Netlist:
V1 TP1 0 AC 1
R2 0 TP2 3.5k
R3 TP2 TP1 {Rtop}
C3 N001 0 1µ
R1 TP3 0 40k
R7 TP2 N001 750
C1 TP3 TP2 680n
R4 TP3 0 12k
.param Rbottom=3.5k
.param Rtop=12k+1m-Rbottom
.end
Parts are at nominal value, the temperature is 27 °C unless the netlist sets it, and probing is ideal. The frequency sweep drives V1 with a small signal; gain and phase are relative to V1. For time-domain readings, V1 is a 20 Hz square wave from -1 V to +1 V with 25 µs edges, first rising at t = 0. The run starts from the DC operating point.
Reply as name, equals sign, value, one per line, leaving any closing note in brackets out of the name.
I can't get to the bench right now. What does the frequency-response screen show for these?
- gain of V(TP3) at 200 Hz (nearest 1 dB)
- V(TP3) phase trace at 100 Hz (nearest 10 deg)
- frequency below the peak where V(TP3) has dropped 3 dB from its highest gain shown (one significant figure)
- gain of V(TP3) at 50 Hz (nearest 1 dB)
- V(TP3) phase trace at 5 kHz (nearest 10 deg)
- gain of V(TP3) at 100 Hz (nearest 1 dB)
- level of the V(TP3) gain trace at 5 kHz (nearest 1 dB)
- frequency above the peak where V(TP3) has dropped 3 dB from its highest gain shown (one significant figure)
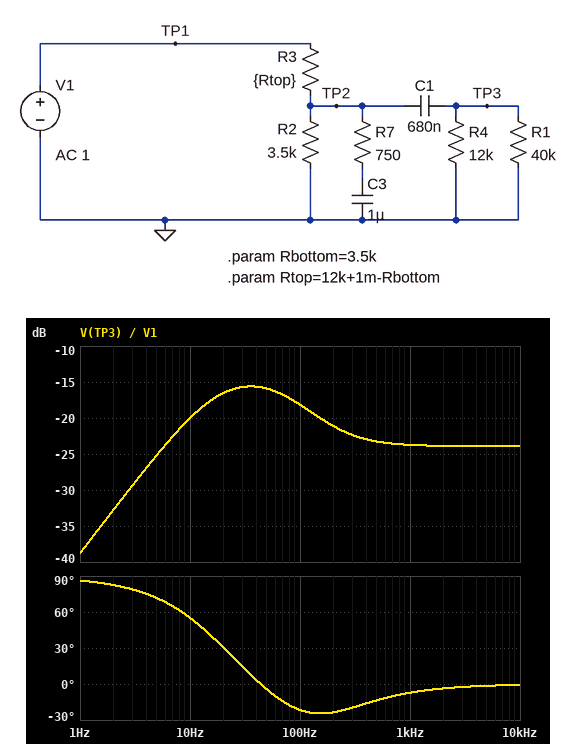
gain of V(TP3) at 200 Hz = -21 dB
V(TP3) phase trace at 100 Hz = -20 deg
frequency below the peak where V(TP3) has dropped 3 dB from its highest gain shown = 10 Hz
gain of V(TP3) at 50 Hz = -16 dB
V(TP3) phase trace at 5 kHz = 0 deg
gain of V(TP3) at 100 Hz = -18 dB
level of the V(TP3) gain trace at 5 kHz = -24 dB
frequency above the peak where V(TP3) has dropped 3 dB from its highest gain shown = 100 Hz
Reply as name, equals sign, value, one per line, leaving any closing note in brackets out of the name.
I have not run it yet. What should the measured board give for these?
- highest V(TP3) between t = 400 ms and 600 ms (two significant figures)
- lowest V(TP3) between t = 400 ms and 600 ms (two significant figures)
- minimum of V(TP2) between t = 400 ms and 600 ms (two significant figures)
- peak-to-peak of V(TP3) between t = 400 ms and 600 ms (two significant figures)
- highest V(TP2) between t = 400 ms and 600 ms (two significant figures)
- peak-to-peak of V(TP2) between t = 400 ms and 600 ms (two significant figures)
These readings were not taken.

highest V(TP3) between t = 400 ms and 600 ms = 240 mV
lowest V(TP3) between t = 400 ms and 600 ms = -240 mV
minimum of V(TP2) between t = 400 ms and 600 ms = -280 mV
peak-to-peak of V(TP3) between t = 400 ms and 600 ms = 480 mV
highest V(TP2) between t = 400 ms and 600 ms = 280 mV
peak-to-peak of V(TP2) between t = 400 ms and 600 ms = 560 mV
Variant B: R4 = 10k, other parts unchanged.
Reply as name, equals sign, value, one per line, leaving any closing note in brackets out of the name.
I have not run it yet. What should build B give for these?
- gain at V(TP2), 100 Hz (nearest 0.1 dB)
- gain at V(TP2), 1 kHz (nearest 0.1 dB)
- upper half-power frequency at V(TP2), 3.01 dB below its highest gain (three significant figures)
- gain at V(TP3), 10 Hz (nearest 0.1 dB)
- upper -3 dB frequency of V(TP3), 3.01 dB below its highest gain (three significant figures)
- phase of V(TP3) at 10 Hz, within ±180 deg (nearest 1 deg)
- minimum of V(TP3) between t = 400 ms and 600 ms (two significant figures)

gain at V(TP2), 100 Hz = -18.0 dB
gain at V(TP2), 1 kHz = -23.8 dB
upper half-power frequency at V(TP2), 3.01 dB below its highest gain = 33.1 Hz
gain at V(TP3), 10 Hz = -21.1 dB
upper -3 dB frequency of V(TP3), 3.01 dB below its highest gain = 121 Hz
phase of V(TP3) at 10 Hz, within ±180 deg = 58 deg
minimum of V(TP3) between t = 400 ms and 600 ms = -230 mV
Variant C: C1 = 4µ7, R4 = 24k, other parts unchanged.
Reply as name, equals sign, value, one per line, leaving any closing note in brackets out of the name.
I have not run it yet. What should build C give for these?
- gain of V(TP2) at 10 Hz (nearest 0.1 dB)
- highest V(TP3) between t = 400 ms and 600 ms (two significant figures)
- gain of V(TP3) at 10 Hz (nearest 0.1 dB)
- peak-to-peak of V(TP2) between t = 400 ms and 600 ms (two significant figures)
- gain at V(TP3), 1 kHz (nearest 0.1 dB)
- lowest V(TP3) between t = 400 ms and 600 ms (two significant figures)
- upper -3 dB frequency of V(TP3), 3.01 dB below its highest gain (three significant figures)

gain of V(TP2) at 10 Hz = -12.1 dB
highest V(TP3) between t = 400 ms and 600 ms = 250 mV
gain of V(TP3) at 10 Hz = -12.4 dB
peak-to-peak of V(TP2) between t = 400 ms and 600 ms = 510 mV
gain at V(TP3), 1 kHz = -23.5 dB
lowest V(TP3) between t = 400 ms and 600 ms = -250 mV
upper -3 dB frequency of V(TP3), 3.01 dB below its highest gain = 64.0 Hz
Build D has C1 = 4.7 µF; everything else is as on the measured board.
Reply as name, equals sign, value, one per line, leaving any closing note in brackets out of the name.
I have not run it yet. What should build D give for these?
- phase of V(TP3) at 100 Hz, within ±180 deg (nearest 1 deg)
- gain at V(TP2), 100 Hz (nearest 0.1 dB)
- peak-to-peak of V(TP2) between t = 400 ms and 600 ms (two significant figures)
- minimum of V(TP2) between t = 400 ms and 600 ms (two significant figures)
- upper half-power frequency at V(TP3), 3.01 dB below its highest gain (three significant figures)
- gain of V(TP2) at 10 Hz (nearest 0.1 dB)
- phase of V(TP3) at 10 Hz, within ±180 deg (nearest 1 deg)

phase of V(TP3) at 100 Hz, within ±180 deg = -32 deg
gain at V(TP2), 100 Hz = -17.8 dB
peak-to-peak of V(TP2) between t = 400 ms and 600 ms = 480 mV
minimum of V(TP2) between t = 400 ms and 600 ms = -240 mV
upper half-power frequency at V(TP3), 3.01 dB below its highest gain = 71.1 Hz
gain of V(TP2) at 10 Hz = -12.8 dB
phase of V(TP3) at 10 Hz, within ±180 deg = 9 deg
